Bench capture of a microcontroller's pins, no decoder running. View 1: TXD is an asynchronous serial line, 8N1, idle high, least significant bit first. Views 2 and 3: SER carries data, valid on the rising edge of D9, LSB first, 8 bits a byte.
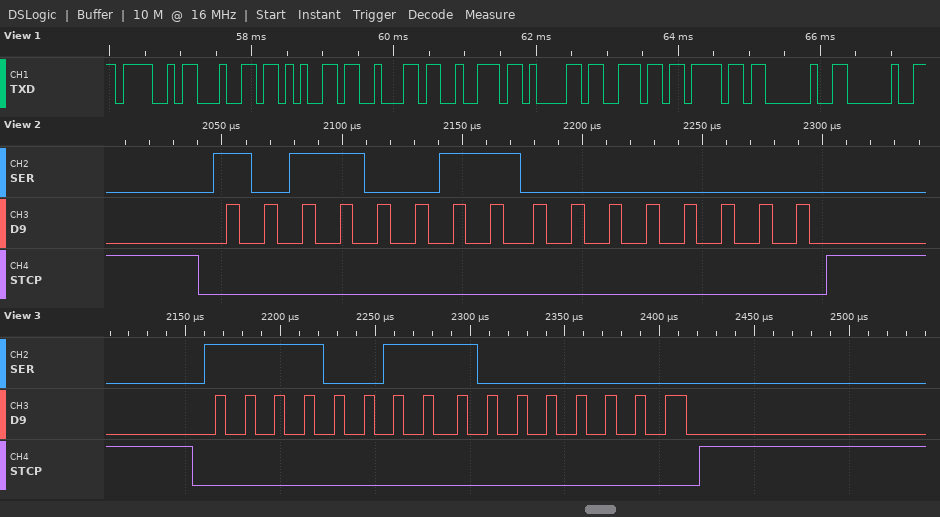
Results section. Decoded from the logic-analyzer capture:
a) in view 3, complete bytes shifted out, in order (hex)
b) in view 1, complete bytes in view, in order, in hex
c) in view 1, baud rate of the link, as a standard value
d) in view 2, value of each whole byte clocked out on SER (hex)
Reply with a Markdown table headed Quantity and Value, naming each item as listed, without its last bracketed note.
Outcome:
| Quantity | Value |
|---|---|
| in view 3, complete bytes shifted out, in order | CF 01 |
| in view 1, complete bytes in view, in order, in hex | 0x4F 0x64 0x65 0x62 0x72 0x61 0x6E 0x6F 0x20 0x20 |
| in view 1, baud rate of the link, as a standard value | 9600 baud |
| in view 2, value of each whole byte clocked out on SER | CD 00 |
